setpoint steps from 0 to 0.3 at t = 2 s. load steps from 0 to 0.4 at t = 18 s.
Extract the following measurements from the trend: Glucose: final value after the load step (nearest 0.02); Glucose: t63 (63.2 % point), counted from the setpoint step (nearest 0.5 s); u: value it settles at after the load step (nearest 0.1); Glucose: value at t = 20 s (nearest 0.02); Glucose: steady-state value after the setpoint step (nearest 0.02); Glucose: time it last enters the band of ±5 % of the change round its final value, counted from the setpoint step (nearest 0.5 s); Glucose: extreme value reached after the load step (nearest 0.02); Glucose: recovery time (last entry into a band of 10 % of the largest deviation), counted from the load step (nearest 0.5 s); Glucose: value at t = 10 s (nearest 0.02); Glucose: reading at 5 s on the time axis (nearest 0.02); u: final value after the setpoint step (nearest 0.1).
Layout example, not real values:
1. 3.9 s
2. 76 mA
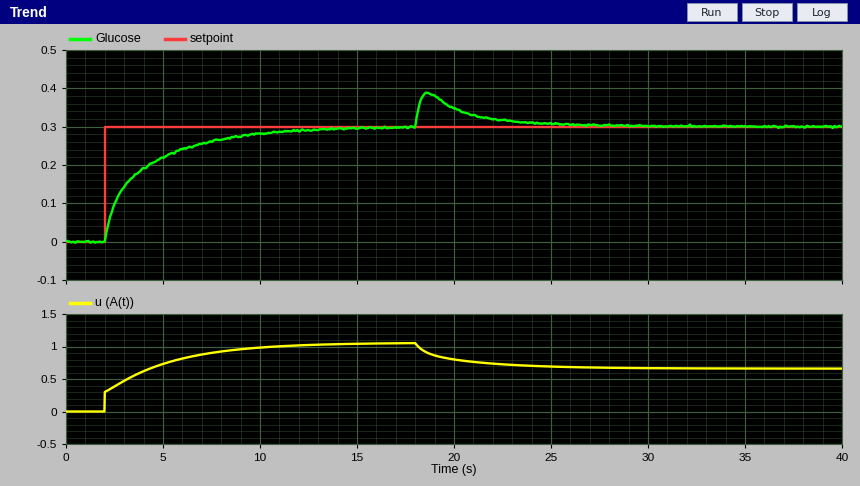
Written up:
1. 0.30
2. 2.0 s
3. 0.7
4. 0.34
5. 0.30
6. 8.5 s
7. 0.38
8. 6.5 s
9. 0.28
10. 0.22
11. 1.1
